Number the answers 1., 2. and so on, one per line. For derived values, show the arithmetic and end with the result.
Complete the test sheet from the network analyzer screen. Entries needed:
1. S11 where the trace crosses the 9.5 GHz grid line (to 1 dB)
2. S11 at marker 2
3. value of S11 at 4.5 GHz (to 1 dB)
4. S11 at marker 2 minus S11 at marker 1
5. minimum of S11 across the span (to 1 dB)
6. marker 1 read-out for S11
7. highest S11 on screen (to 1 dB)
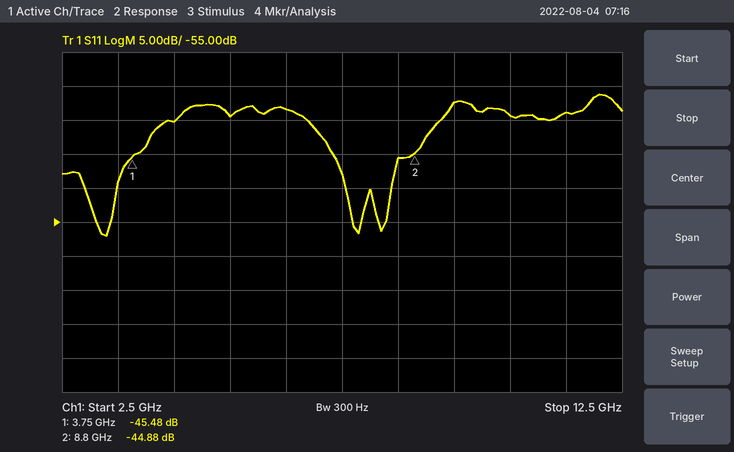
1. -37 dB
2. -44.88 dB
3. -40 dB
4. -44.88 − (-45.48) = 0.60 dB
5. -57 dB
6. -45.48 dB
7. -36 dB
